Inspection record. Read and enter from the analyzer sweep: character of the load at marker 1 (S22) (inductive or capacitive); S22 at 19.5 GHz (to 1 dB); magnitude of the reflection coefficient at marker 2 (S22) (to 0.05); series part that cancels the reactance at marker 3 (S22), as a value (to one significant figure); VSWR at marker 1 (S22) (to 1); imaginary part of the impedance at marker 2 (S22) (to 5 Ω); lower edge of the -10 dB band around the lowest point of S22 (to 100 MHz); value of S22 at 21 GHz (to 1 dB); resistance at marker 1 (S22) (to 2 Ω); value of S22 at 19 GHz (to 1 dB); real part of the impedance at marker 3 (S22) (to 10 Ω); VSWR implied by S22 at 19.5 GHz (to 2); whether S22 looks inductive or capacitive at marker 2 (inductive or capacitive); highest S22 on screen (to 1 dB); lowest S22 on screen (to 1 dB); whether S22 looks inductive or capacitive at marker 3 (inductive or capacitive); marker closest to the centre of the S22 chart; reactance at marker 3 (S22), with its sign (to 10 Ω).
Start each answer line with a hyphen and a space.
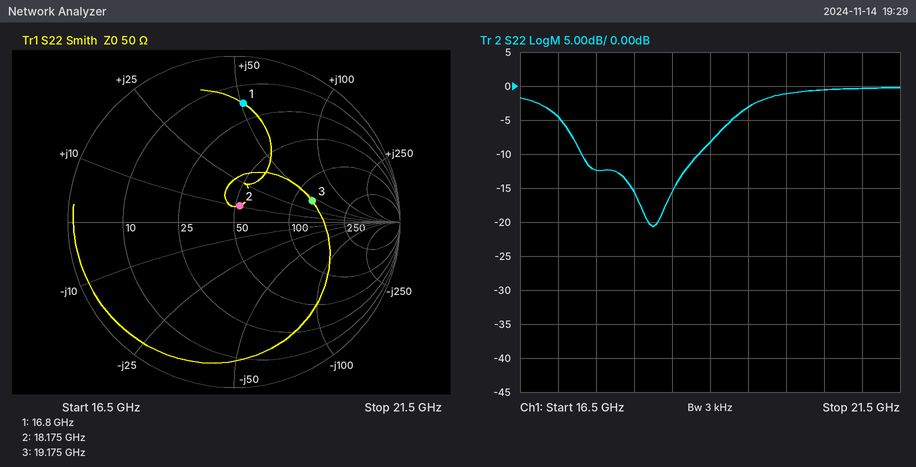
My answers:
- inductive
- -3 dB
- 0.10
- 200 fF
- 6
- +10 Ω
- 17.3 GHz
- 0 dB
- 18 Ω
- -8 dB
- 130 Ω
- 6
- inductive
- 0 dB
- -21 dB
- inductive
- marker 2
- +40 Ω
